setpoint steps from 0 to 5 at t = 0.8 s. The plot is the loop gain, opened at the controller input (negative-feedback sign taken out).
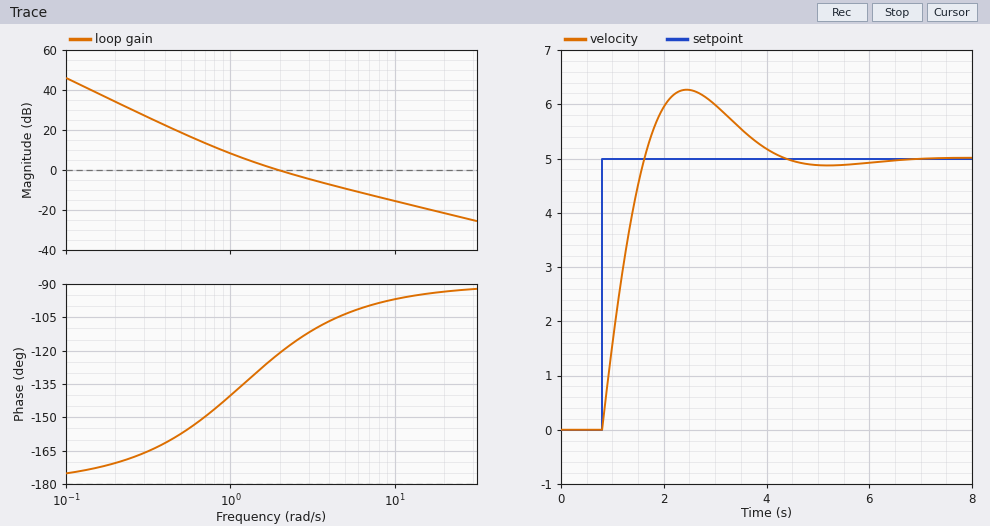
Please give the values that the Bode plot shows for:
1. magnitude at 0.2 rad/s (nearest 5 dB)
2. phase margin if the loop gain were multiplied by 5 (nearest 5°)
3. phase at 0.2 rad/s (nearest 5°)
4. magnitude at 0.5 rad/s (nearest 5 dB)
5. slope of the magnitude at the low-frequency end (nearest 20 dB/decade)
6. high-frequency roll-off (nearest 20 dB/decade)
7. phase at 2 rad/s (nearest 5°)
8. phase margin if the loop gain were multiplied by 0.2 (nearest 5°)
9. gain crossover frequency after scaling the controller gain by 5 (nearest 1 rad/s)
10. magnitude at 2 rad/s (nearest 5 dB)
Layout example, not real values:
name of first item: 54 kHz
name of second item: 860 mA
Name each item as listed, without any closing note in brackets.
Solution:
magnitude at 0.2 rad/s: 35 dB
phase margin if the loop gain were multiplied by 5: 80°
phase at 0.2 rad/s: -170°
magnitude at 0.5 rad/s: 20 dB
slope of the magnitude at the low-frequency end: -40 dB/decade
high-frequency roll-off: -20 dB/decade
phase at 2 rad/s: -120°
phase margin if the loop gain were multiplied by 0.2: 30°
gain crossover frequency after scaling the controller gain by 5: 8 rad/s
magnitude at 2 rad/s: 0 dB
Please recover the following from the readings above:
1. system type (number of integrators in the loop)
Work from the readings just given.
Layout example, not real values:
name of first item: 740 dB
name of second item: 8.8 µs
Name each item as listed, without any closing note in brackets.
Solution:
system type: 2
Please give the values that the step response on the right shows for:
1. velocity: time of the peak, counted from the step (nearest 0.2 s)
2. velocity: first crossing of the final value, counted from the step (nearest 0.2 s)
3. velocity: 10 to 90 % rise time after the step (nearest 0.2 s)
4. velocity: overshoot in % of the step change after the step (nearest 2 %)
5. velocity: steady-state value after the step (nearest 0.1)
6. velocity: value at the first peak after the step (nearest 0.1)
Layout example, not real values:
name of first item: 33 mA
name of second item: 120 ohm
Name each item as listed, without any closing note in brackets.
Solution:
velocity: time of the peak, counted from the step: 1.6 s
velocity: first crossing of the final value, counted from the step: 0.8 s
velocity: 10 to 90 % rise time after the step: 0.6 s
velocity: overshoot in % of the step change after the step: 26 %
velocity: steady-state value after the step: 5.0
velocity: value at the first peak after the step: 6.3
